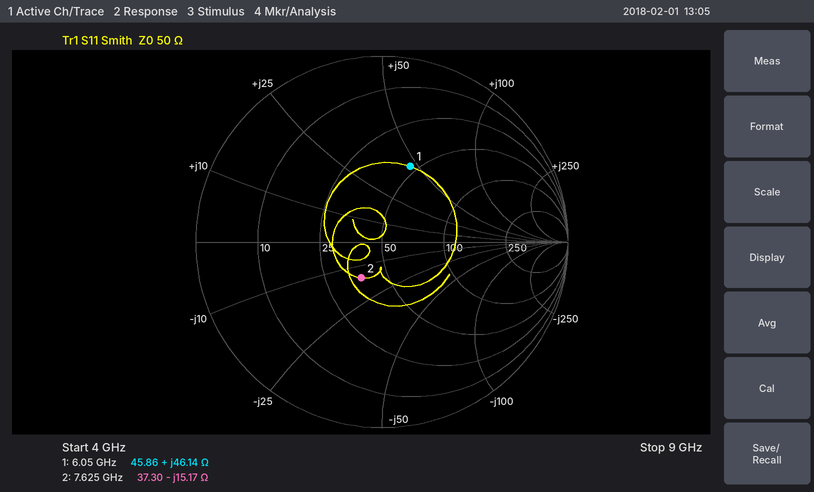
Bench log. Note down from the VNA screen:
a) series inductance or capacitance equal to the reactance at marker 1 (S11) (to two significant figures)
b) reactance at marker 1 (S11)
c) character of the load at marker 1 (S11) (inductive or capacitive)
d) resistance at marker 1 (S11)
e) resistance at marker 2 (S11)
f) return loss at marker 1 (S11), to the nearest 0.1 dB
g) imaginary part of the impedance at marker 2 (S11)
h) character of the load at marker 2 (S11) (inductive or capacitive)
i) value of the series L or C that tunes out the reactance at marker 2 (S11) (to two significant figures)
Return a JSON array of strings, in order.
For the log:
["1.2 nH", "+46.14 Ω", "inductive", "45.86 Ω", "37.30 Ω", "7.2 dB", "-15.17 Ω", "capacitive", "320 pH"]
